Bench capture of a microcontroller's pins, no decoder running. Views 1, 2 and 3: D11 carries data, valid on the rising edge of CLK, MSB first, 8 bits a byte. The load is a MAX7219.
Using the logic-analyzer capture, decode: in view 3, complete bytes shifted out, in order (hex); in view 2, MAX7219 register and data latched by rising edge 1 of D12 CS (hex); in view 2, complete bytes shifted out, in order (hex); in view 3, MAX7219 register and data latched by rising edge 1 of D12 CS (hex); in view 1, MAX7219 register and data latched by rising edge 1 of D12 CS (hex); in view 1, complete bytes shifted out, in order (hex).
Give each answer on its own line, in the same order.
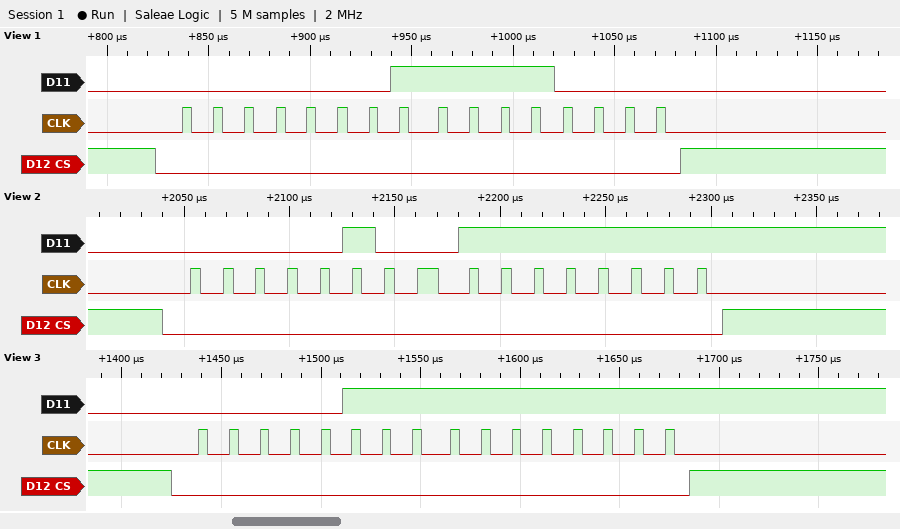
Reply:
07 FF
register 0x4, data 0xFF
04 FF
register 0x7, data 0xFF
register 0x1, data 0xF0
01 F0
